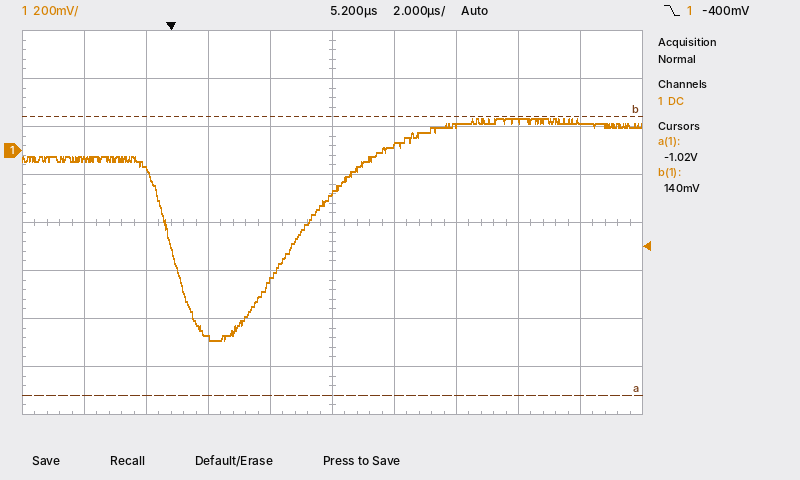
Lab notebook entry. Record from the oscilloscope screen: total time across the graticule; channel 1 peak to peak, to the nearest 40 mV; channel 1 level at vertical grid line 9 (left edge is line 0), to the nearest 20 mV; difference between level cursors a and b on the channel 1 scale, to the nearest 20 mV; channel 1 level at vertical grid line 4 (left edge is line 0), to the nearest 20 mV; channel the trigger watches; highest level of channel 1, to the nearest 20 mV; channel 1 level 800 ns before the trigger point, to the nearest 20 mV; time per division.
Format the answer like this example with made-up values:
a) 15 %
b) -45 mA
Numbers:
a) 20 µs
b) 920 mV
c) 120 mV
d) 1.16 V
e) -540 mV
f) channel 1
g) 140 mV
h) -80 mV
i) 2 µs
